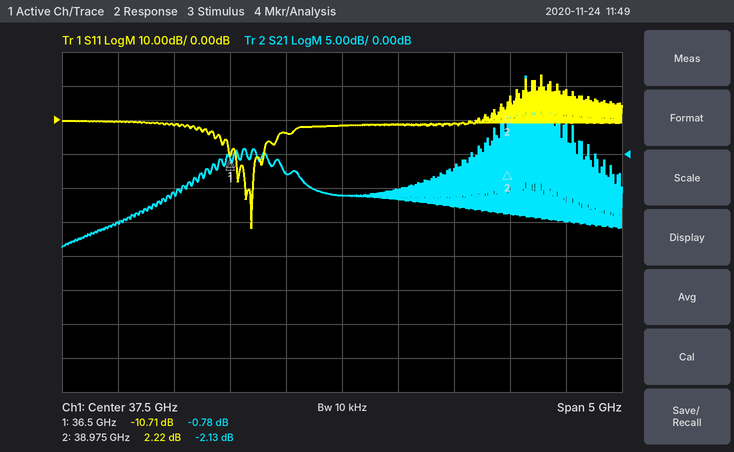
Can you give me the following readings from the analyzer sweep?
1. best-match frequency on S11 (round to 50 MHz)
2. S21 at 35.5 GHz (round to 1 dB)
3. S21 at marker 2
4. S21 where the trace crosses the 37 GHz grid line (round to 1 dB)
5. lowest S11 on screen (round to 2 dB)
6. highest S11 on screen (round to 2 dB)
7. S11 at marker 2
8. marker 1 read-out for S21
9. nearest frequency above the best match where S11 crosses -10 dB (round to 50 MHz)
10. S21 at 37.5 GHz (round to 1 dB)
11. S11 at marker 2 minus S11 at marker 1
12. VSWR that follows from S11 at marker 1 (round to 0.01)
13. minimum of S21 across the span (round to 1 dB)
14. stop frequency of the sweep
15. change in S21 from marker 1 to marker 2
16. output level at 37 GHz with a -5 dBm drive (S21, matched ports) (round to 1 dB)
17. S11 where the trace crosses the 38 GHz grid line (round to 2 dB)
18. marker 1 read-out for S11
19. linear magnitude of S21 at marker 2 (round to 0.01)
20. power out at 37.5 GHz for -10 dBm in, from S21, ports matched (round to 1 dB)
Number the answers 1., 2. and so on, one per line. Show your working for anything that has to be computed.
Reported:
1. 36.70 GHz
2. -10 dB
3. -2.13 dB
4. -3 dB
5. -32 dB
6. 14 dB
7. 2.22 dB
8. -0.78 dB
9. 36.80 GHz
10. -6 dB
11. 2.22 − (-10.71) = 12.93 dB
12. (1 + 0.2914)/(1 − 0.2914) ≈ 1.82
13. -14 dB
14. 40 GHz
15. -2.13 − (-0.78) = -1.35 dB
16. -5 dBm + (-3 dB) = -8 dBm
17. -2 dB
18. -10.71 dB
19. 10^(-2.13/20) ≈ 0.78
20. -10 dBm + (-6 dB) = -16 dBm
